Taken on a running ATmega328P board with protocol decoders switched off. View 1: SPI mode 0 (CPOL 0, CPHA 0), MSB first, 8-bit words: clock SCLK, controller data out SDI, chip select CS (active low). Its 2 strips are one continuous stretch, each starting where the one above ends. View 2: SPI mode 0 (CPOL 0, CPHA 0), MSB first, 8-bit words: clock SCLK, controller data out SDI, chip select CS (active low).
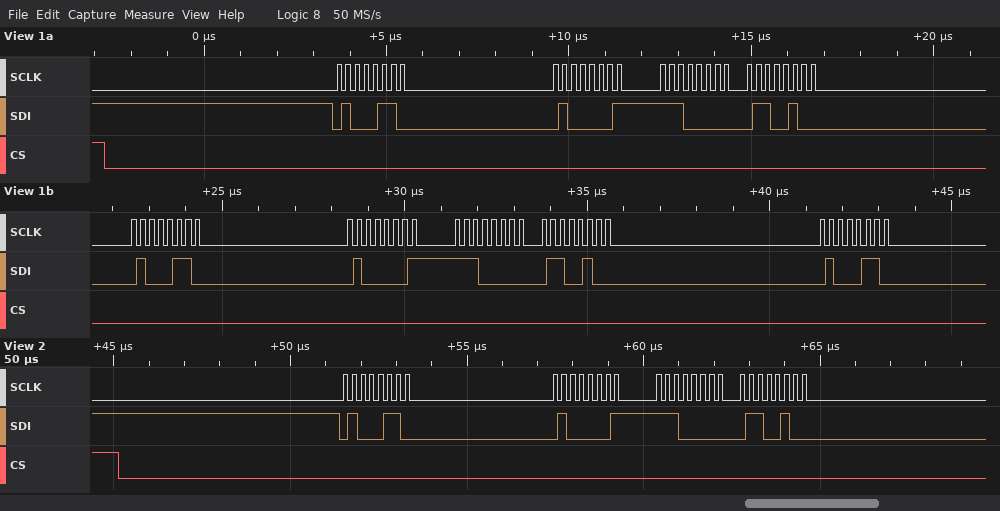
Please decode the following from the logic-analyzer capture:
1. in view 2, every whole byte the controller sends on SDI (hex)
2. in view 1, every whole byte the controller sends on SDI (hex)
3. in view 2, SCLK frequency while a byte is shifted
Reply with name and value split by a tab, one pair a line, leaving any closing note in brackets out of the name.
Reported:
in view 2, every whole byte the controller sends on SDI	0x46 0x41 0xE0 0x64
in view 1, every whole byte the controller sends on SDI	46 41 E0 64 46 41 E0 64 46
in view 2, SCLK frequency while a byte is shifted	4 MHz
